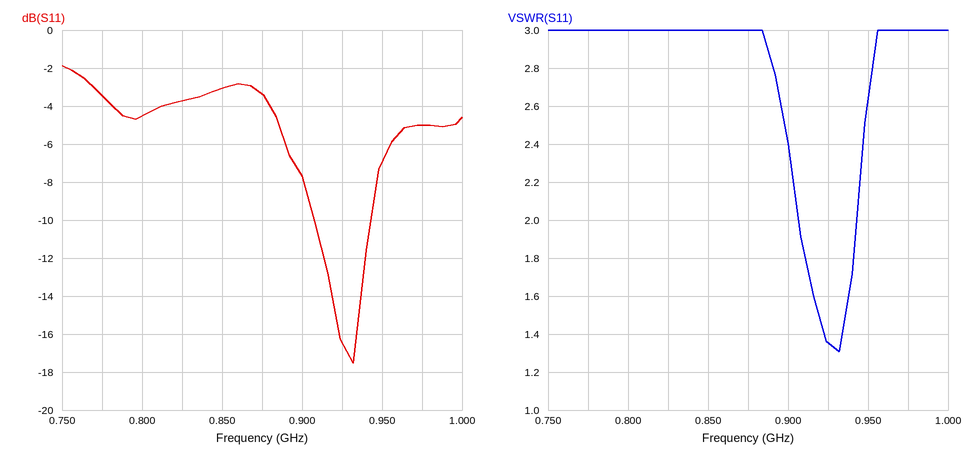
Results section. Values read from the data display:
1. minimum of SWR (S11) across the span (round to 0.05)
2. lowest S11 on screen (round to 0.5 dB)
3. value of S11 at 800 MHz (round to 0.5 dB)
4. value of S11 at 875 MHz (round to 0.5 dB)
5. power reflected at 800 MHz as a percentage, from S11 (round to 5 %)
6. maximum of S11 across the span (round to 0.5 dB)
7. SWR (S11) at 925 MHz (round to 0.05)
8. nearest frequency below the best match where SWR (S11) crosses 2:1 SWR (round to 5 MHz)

1.30
-17.5 dB
-4.5 dB
-3.5 dB
35 %
-2.0 dB
1.35
905 MHz
